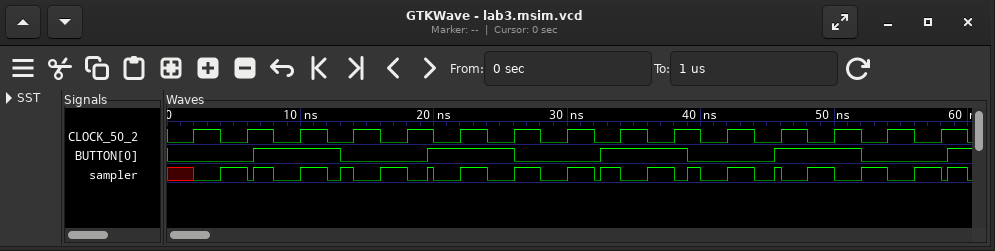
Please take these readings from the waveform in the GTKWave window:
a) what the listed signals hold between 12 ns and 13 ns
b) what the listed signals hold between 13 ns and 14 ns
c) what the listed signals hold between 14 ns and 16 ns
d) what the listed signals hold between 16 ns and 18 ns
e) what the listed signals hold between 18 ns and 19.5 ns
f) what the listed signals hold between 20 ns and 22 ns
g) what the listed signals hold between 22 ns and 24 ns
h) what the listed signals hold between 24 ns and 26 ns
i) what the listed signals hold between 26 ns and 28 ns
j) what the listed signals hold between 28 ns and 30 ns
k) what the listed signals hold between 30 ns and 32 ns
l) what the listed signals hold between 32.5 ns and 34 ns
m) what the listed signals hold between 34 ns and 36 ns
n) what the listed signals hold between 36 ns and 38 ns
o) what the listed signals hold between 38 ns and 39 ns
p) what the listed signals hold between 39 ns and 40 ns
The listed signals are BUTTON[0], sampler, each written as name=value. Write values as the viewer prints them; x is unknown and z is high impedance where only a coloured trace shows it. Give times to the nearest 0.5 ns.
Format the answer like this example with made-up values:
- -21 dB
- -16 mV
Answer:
- BUTTON[0]=1, sampler=0
- BUTTON[0]=0, sampler=1
- BUTTON[0]=0, sampler=0
- BUTTON[0]=0, sampler=1
- BUTTON[0]=0, sampler=0
- BUTTON[0]=1, sampler=0
- BUTTON[0]=1, sampler=1
- BUTTON[0]=1, sampler=0
- BUTTON[0]=0, sampler=1
- BUTTON[0]=0, sampler=0
- BUTTON[0]=0, sampler=1
- BUTTON[0]=1, sampler=1
- BUTTON[0]=1, sampler=0
- BUTTON[0]=1, sampler=1
- BUTTON[0]=1, sampler=0
- BUTTON[0]=0, sampler=1
